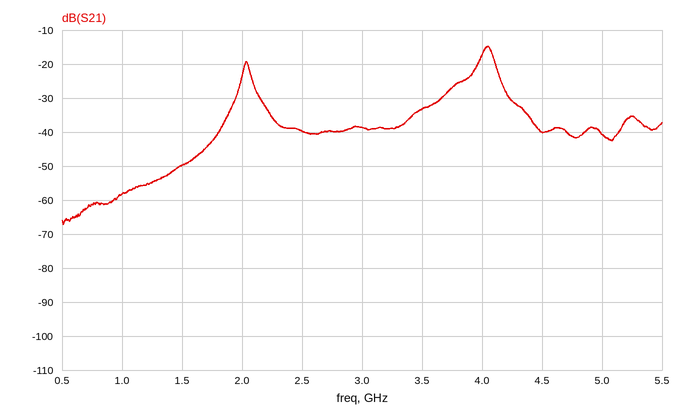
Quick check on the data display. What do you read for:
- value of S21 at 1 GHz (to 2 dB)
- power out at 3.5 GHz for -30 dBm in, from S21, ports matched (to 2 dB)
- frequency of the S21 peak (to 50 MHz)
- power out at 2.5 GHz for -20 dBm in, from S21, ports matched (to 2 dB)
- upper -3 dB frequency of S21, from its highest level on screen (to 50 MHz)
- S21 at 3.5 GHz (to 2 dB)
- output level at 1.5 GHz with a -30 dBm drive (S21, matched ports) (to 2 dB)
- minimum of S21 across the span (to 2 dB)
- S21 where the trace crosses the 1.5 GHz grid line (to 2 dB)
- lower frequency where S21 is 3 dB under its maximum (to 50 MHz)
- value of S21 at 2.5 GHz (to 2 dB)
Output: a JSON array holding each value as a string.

["-58 dB", "-64 dBm", "4.05 GHz", "-60 dBm", "4.10 GHz", "-34 dB", "-80 dBm", "-68 dB", "-50 dB", "4.00 GHz", "-40 dB"]
